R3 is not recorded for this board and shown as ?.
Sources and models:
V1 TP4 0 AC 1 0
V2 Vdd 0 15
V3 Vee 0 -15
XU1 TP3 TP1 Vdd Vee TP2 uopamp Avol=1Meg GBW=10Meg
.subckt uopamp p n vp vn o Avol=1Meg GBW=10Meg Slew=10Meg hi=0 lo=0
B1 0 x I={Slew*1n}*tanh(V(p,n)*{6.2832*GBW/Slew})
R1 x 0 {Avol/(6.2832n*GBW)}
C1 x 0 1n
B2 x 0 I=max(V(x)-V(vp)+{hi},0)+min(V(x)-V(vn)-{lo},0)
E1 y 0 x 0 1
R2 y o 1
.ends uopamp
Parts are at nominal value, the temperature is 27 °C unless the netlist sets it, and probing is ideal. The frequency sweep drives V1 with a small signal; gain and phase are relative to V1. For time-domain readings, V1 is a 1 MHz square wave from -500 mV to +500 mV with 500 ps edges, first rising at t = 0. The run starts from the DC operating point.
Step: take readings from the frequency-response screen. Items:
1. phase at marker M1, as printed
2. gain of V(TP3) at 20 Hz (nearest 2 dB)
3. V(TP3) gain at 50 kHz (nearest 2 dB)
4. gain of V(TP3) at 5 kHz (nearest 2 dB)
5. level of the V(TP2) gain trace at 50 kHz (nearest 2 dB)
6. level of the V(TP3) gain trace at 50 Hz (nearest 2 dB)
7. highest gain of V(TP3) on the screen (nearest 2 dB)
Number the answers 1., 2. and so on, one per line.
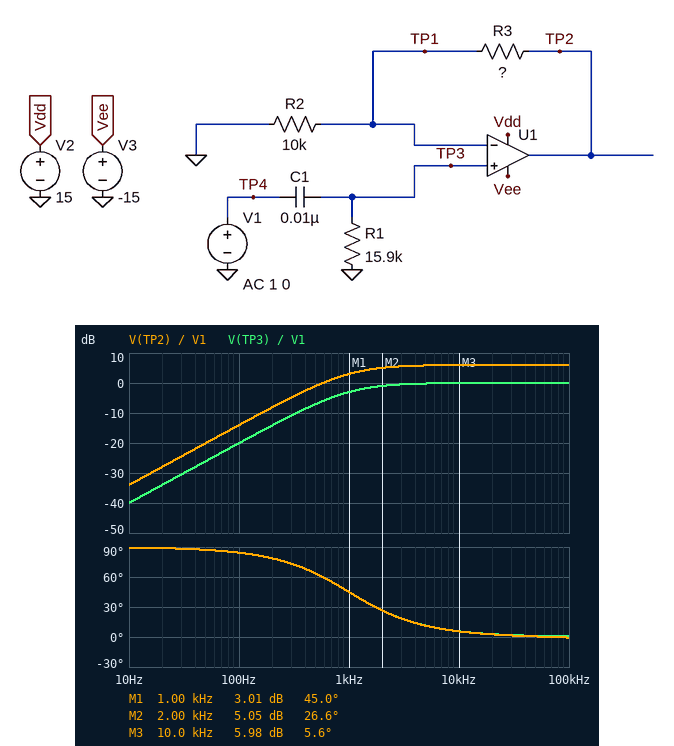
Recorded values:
1. 45.0 deg
2. -34 dB
3. 0 dB
4. 0 dB
5. 6 dB
6. -26 dB
7. 0 dB
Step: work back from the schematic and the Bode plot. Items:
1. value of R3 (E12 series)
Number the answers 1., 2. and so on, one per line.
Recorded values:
1. 10 kΩ
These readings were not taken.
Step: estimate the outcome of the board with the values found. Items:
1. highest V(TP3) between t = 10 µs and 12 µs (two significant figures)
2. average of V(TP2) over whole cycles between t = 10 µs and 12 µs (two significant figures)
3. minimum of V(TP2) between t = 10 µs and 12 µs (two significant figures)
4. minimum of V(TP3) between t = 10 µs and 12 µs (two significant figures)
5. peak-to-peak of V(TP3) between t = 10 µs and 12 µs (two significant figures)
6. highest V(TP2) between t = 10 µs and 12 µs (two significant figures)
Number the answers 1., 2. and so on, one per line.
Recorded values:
1. 970 mV
2. 930 mV
3. -73 mV
4. -36 mV
5. 1.0 V
6. 1.9 V
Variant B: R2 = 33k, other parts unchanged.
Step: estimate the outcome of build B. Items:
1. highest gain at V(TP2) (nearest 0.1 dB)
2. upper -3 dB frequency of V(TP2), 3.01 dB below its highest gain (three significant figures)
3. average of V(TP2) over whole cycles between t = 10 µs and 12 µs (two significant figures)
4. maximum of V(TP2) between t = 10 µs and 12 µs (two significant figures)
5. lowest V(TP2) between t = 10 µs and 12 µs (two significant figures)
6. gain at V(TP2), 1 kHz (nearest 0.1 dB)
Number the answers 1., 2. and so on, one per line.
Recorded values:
1. 2.3 dB
2. 7.68 MHz
3. 610 mV
4. 1.3 V
5. -47 mV
6. -0.7 dB
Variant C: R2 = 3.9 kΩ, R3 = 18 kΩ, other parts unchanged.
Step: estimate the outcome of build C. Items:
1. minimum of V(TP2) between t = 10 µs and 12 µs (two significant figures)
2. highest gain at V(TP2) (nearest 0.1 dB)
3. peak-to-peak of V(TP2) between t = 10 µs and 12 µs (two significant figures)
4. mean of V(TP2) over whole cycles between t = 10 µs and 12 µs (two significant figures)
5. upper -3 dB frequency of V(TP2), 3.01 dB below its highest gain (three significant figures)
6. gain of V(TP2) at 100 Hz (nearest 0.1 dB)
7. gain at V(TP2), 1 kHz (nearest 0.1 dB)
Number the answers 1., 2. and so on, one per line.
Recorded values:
1. 290 mV
2. 15.0 dB
3. 4.7 V
4. 2.6 V
5. 1.78 MHz
6. -5.1 dB
7. 12.0 dB
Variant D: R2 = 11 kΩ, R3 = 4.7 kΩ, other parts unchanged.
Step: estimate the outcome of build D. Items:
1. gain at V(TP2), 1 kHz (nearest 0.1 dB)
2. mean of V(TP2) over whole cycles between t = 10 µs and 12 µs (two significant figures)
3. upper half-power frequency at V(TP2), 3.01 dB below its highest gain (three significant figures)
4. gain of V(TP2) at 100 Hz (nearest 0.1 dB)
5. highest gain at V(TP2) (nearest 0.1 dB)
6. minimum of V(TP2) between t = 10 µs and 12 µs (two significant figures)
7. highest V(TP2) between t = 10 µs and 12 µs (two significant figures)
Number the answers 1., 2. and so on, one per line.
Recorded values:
1. 0.1 dB
2. 670 mV
3. 7.01 MHz
4. -17.0 dB
5. 3.1 dB
6. -52 mV
7. 1.4 V
